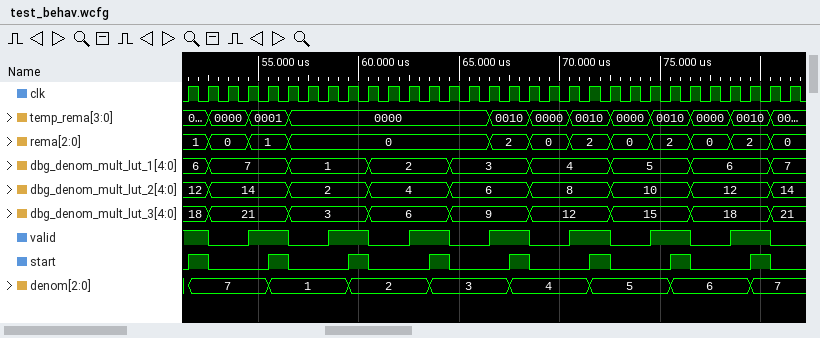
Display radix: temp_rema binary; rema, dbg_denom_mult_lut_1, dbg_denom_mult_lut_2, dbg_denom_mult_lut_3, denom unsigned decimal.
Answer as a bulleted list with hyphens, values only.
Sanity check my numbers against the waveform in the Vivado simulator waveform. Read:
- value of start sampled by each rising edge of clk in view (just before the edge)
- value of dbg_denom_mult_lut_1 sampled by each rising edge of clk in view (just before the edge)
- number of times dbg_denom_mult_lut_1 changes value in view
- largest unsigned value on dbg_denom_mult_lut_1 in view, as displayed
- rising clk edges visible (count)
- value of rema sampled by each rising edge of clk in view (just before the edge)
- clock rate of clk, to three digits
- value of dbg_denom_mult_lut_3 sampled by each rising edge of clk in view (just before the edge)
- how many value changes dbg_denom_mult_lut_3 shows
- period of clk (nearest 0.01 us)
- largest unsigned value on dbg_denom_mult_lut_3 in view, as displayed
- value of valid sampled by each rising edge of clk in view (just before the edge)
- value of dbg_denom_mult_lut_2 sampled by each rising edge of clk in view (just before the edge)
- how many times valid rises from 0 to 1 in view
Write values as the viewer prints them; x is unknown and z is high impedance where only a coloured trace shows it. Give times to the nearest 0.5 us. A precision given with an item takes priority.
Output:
- 0 1 0 0 0 1 0 0 0 1 0 0 0 1 0 0 0 1 0 0 0 1 0 0 0 1 0 0 0 1 0
- 6, 6, 7, 7, 7, 7, 1, 1, 1, 1, 2, 2, 2, 2, 3, 3, 3, 3, 4, 4, 4, 4, 5, 5, 5, 5, 6, 6, 6, 6, 7
- 8
- 7
- 31
- 1, 1, 0, 0, 1, 1, 0, 0, 0, 0, 0, 0, 0, 0, 0, 0, 2, 2, 0, 0, 2, 2, 0, 0, 2, 2, 0, 0, 2, 2, 0
- 1.00 MHz
- 18, 18, 21, 21, 21, 21, 3, 3, 3, 3, 6, 6, 6, 6, 9, 9, 9, 9, 12, 12, 12, 12, 15, 15, 15, 15, 18, 18, 18, 18, 21
- 8
- 1 us
- 21
- 1 1 0 0 1 1 0 0 1 1 0 0 1 1 0 0 1 1 0 0 1 1 0 0 1 1 0 0 1 1 0
- 12, 12, 14, 14, 14, 14, 2, 2, 2, 2, 4, 4, 4, 4, 6, 6, 6, 6, 8, 8, 8, 8, 10, 10, 10, 10, 12, 12, 12, 12, 14
- 7
